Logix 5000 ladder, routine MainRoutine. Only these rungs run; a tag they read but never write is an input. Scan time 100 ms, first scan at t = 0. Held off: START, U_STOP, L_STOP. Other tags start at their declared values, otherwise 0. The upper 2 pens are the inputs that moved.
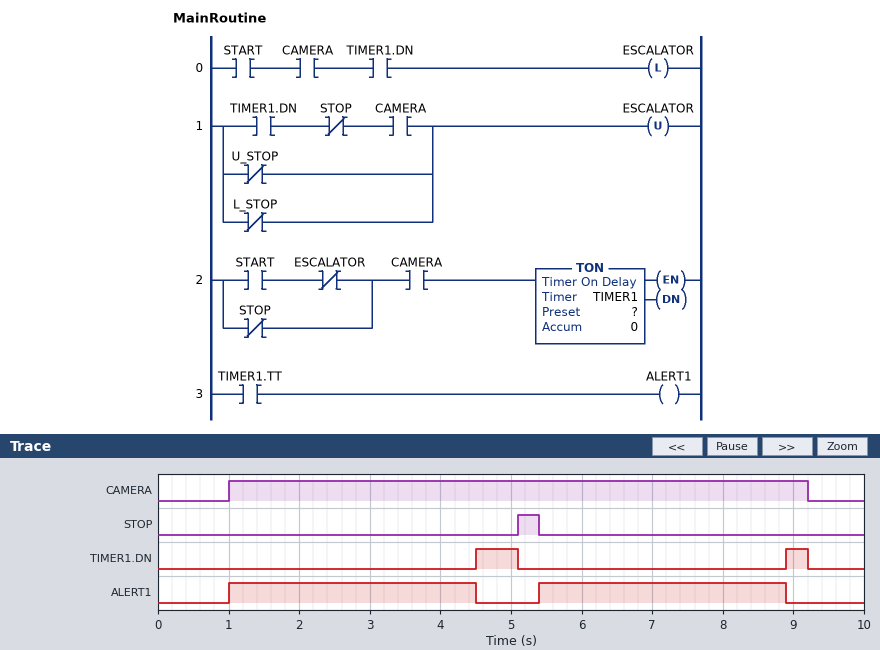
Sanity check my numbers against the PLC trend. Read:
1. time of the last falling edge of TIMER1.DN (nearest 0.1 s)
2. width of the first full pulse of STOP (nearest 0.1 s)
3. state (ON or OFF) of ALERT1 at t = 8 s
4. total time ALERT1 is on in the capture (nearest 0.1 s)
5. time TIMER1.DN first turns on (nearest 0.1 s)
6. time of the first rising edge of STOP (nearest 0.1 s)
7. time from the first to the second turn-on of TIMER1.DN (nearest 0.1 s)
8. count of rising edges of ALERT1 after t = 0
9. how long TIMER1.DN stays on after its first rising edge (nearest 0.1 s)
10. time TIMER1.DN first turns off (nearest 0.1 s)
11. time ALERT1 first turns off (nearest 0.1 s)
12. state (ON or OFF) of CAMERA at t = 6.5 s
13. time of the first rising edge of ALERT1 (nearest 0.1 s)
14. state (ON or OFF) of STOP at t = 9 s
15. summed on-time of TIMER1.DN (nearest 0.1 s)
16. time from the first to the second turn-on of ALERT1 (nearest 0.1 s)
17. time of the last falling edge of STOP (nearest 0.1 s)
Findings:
9.2 s
0.3 s
ON
7.0 s
4.5 s
5.1 s
4.4 s
2
0.6 s
5.1 s
4.5 s
ON
1.0 s
OFF
0.9 s
4.4 s
5.4 s
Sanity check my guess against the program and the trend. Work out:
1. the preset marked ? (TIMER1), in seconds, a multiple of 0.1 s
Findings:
3.5 s
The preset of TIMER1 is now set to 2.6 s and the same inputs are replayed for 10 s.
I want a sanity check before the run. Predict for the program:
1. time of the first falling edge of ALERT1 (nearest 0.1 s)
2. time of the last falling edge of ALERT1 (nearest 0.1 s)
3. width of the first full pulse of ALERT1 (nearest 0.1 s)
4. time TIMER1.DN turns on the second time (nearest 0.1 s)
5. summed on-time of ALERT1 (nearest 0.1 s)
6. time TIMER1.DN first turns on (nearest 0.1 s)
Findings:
3.6 s
8.0 s
2.6 s
8.0 s
5.2 s
3.6 s
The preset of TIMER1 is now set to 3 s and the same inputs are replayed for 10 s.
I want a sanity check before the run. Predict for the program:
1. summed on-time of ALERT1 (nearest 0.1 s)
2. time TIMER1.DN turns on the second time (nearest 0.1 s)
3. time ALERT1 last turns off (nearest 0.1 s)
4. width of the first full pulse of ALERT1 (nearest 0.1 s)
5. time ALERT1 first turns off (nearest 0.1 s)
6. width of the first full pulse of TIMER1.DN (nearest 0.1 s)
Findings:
6.0 s
8.4 s
8.4 s
3.0 s
4.0 s
1.1 s
